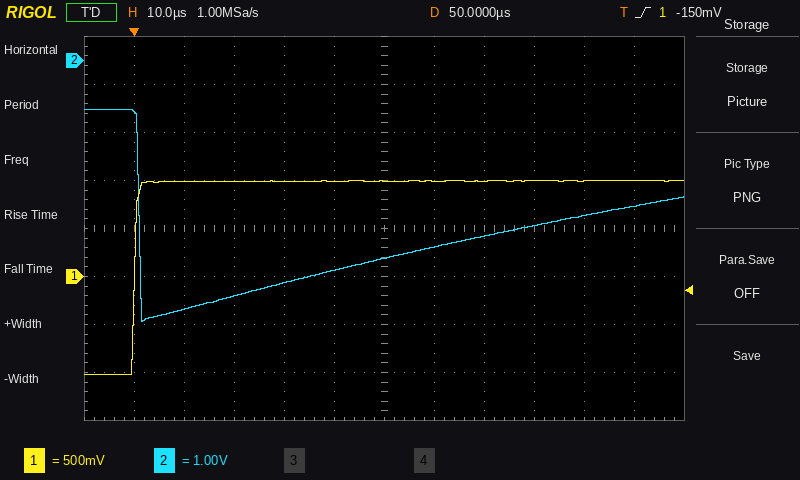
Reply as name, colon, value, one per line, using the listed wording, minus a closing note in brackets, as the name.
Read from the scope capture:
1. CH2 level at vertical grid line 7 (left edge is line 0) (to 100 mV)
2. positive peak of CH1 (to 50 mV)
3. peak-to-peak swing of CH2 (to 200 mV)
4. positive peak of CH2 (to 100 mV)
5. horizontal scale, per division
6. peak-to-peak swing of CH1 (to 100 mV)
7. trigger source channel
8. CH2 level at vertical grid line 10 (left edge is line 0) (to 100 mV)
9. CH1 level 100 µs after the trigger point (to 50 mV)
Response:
CH2 level at vertical grid line 7 (left edge is line 0): -3.9 V
positive peak of CH1: 1.00 V
peak-to-peak swing of CH2: 4.4 V
positive peak of CH2: -1.0 V
horizontal scale, per division: 10 µs
peak-to-peak swing of CH1: 2.00 V
trigger source channel: CH1
CH2 level at vertical grid line 10 (left edge is line 0): -3.2 V
CH1 level 100 µs after the trigger point: 1.00 V
